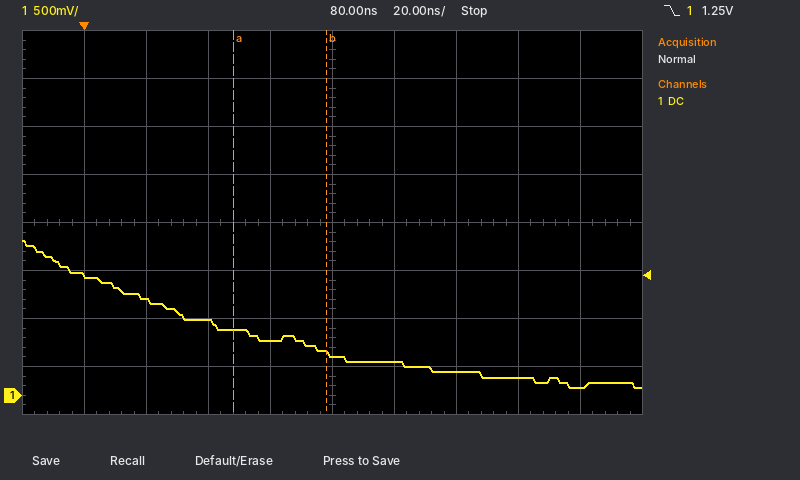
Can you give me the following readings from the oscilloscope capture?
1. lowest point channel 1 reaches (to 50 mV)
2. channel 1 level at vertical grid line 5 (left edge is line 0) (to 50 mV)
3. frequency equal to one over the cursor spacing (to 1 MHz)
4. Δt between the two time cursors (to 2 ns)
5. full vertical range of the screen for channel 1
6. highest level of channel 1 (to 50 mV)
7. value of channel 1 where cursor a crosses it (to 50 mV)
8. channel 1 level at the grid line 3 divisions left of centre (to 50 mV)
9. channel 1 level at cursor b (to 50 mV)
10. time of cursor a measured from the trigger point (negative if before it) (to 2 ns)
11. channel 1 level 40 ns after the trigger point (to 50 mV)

100 mV
400 mV
33 MHz
30 ns
4 V
1.60 V
700 mV
1.00 V
450 mV
+48 ns
800 mV
